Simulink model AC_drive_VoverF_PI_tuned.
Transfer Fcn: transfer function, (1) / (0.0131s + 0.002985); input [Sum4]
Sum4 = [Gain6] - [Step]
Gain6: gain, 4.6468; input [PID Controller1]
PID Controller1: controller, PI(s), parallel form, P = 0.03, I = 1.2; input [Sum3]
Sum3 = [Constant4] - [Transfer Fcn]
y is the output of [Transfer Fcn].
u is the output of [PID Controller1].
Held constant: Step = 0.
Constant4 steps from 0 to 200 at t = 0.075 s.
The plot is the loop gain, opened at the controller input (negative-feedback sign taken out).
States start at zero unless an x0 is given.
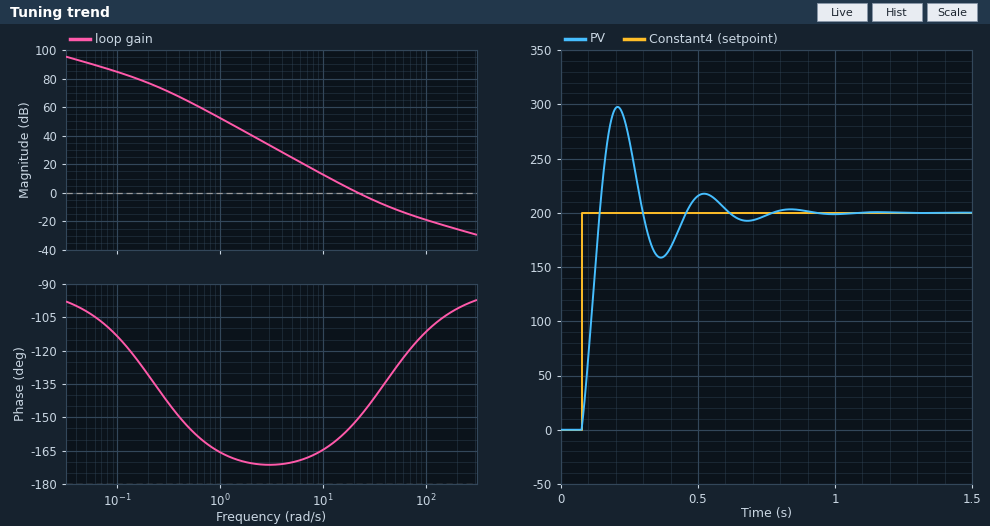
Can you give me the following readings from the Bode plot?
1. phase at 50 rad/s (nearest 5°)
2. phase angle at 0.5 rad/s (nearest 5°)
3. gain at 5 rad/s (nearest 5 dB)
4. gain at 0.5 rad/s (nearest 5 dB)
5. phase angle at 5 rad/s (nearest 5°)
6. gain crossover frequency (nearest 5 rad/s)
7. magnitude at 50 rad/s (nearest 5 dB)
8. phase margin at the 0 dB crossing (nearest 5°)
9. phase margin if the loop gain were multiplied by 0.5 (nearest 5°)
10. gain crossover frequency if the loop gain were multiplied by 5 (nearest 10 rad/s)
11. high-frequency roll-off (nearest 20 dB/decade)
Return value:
-130°
-155°
25 dB
65 dB
-170°
20 rad/s
-10 dB
30°
20°
60 rad/s
-20 dB/decade
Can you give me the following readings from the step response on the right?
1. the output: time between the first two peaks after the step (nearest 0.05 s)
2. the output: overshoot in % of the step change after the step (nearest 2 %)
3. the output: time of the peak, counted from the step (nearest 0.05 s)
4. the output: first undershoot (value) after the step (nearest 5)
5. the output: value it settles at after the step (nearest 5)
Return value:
0.30 s
48 %
0.15 s
160
200
